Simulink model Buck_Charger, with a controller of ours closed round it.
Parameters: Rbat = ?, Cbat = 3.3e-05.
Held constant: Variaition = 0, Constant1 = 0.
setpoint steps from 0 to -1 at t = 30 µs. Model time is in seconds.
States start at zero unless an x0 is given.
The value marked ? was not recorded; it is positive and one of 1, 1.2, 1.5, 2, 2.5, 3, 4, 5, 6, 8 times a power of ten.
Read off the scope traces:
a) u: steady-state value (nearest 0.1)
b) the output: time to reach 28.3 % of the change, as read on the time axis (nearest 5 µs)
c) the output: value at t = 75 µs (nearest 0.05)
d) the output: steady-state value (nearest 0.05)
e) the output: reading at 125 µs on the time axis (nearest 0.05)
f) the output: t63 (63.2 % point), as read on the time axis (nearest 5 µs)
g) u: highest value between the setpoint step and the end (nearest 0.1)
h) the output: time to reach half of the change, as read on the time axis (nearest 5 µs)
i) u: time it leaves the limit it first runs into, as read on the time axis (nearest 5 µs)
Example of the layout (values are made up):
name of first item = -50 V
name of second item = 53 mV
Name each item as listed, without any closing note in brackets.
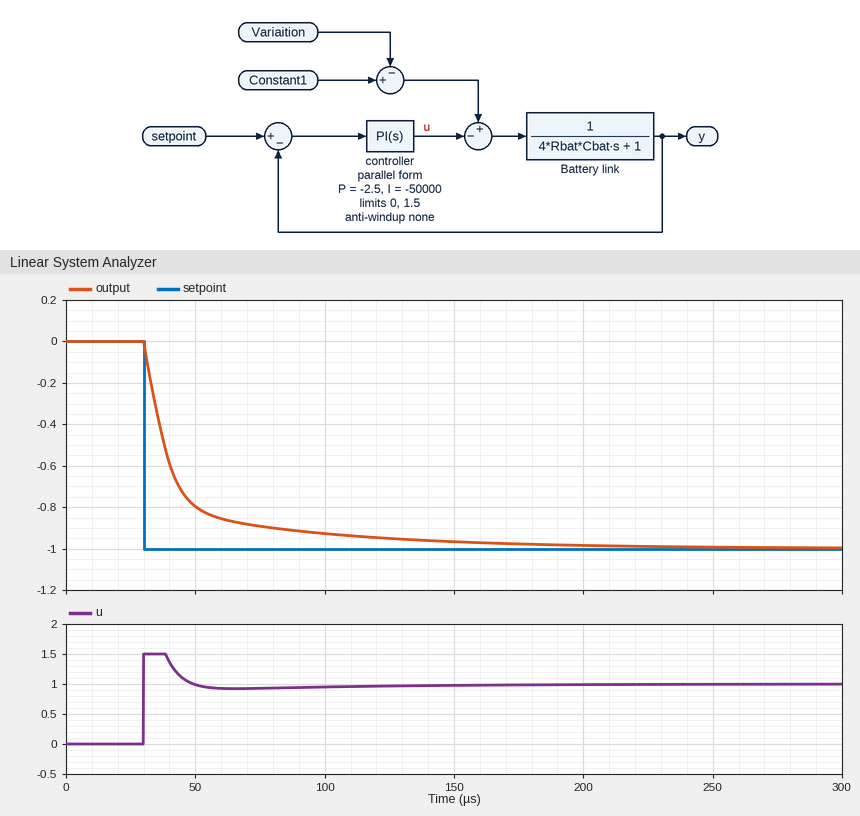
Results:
u: steady-state value = 1.0
the output: time to reach 28.3 % of the change, as read on the time axis = 35 µs
the output: value at t = 75 µs = -0.90
the output: steady-state value = -1.00
the output: reading at 125 µs on the time axis = -0.95
the output: t63 (63.2 % point), as read on the time axis = 40 µs
u: highest value between the setpoint step and the end = 1.5
the output: time to reach half of the change, as read on the time axis = 40 µs
u: time it leaves the limit it first runs into, as read on the time axis = 40 µs
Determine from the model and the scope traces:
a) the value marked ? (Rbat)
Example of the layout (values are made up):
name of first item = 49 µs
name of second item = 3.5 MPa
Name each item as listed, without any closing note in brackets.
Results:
the value marked ? = 0.15
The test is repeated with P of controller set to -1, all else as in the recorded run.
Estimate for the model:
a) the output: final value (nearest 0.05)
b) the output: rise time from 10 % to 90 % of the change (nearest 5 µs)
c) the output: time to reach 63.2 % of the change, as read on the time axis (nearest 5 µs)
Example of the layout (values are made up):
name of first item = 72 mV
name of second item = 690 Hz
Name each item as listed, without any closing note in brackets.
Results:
the output: final value = -1.00
the output: rise time from 10 % to 90 % of the change = 45 µs
the output: time to reach 63.2 % of the change, as read on the time axis = 50 µs
